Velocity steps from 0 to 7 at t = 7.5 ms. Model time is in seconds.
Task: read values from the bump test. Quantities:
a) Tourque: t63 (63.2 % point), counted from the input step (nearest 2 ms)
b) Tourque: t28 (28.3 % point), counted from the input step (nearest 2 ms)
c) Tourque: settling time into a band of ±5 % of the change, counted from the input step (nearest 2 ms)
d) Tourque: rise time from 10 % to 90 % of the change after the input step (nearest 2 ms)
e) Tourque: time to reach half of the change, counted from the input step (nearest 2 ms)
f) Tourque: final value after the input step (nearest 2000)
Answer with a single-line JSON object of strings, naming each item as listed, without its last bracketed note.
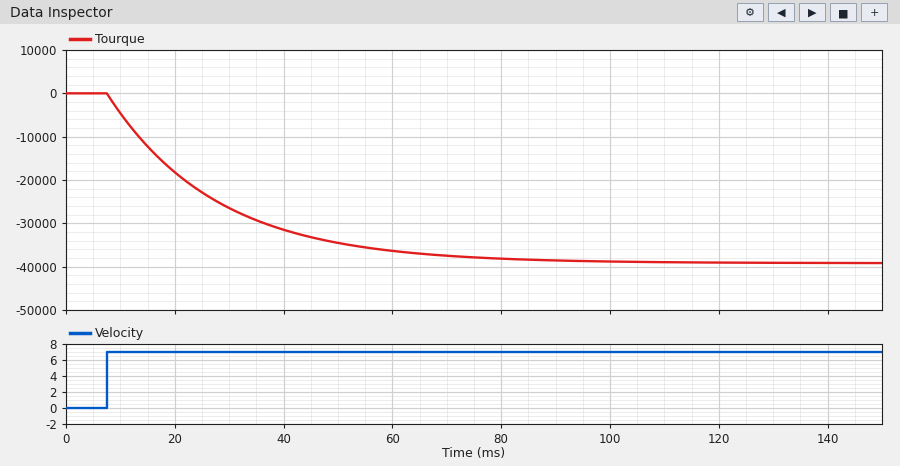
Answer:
{"Tourque: t63 (63.2 % point), counted from the input step": "20 ms", "Tourque: t28 (28.3 % point), counted from the input step": "6 ms", "Tourque: settling time into a band of ±5 % of the change, counted from the input step": "60 ms", "Tourque: rise time from 10 % to 90 % of the change after the input step": "44 ms", "Tourque: time to reach half of the change, counted from the input step": "14 ms", "Tourque: final value after the input step": "-40000"}
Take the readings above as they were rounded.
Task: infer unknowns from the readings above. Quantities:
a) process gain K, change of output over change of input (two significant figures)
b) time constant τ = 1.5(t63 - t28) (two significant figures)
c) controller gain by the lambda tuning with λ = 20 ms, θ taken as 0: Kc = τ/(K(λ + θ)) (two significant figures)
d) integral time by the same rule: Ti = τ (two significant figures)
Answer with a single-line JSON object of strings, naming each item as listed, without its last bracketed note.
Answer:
{"process gain K, change of output over change of input": "-5700", "time constant τ = 1.5(t63 - t28)": "21 ms", "controller gain by the lambda tuning with λ = 20 ms, θ taken as 0: Kc = τ/(K(λ + θ))": "-0.00018", "integral time by the same rule: Ti = τ": "21 ms"}
